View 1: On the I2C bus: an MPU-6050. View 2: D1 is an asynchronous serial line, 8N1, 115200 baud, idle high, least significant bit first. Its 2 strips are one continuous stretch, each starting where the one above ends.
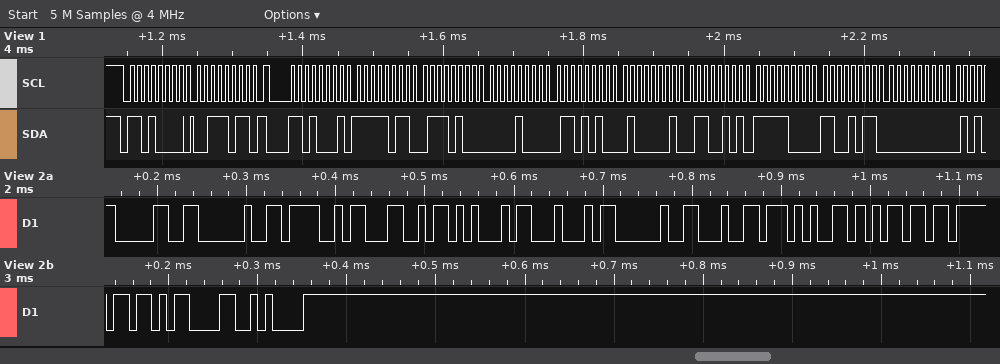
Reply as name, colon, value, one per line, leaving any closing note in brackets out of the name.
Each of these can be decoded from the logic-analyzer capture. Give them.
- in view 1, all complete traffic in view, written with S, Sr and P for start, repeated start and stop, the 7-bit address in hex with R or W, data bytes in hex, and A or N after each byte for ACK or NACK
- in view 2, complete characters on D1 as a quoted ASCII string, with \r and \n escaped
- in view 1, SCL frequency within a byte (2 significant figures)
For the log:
in view 1, all complete traffic in view, written with S, Sr and P for start, repeated start and stop, the 7-bit address in hex with R or W, data bytes in hex, and A or N after each byte for ACK or NACK: S 68W A 3B A Sr 68R A FB A 74 A 08 A 6A A 41 A 65 A F8 A CB A 00 A
in view 2, complete characters on D1 as a quoted ASCII string, with \r and \n escaped: "0 OLED demo\r\n"
in view 1, SCL frequency within a byte: 100 kHz
